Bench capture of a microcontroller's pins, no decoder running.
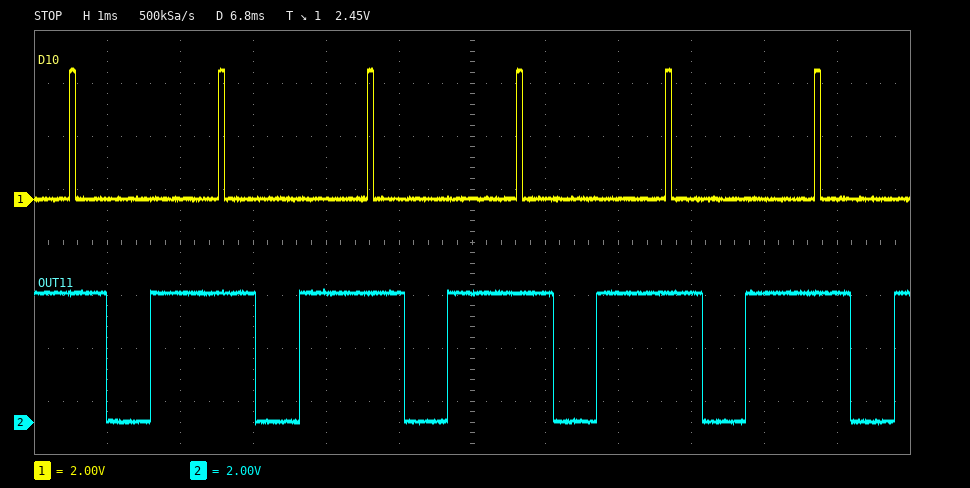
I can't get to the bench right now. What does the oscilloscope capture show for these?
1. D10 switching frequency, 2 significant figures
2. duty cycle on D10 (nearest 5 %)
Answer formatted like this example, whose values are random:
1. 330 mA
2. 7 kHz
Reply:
1. 490 Hz
2. 5 %
